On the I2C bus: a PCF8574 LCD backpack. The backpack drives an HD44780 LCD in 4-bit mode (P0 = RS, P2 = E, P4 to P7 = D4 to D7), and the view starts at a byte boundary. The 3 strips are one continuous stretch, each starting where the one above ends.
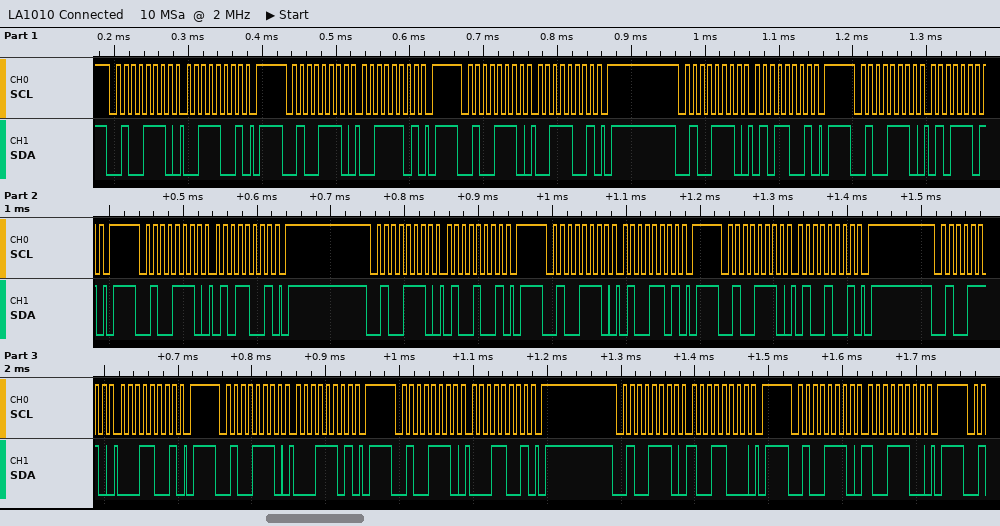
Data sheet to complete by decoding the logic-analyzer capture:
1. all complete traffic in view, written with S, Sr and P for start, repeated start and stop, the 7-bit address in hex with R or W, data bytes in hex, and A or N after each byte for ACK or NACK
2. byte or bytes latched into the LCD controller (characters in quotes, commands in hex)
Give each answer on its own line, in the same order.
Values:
S 27W A 39 A P S 27W A 3D A P S 27W A 39 A P S 27W A 59 A P S 27W A 5D A P S 27W A 59 A P S 27W A 49 A P S 27W A 4D A P S 27W A 49 A P S 27W A 19 A P S 27W A 1D A P S 27W A 19 A P S 27W A 98 A P S 27W A 9C A P
'5' 'A'
